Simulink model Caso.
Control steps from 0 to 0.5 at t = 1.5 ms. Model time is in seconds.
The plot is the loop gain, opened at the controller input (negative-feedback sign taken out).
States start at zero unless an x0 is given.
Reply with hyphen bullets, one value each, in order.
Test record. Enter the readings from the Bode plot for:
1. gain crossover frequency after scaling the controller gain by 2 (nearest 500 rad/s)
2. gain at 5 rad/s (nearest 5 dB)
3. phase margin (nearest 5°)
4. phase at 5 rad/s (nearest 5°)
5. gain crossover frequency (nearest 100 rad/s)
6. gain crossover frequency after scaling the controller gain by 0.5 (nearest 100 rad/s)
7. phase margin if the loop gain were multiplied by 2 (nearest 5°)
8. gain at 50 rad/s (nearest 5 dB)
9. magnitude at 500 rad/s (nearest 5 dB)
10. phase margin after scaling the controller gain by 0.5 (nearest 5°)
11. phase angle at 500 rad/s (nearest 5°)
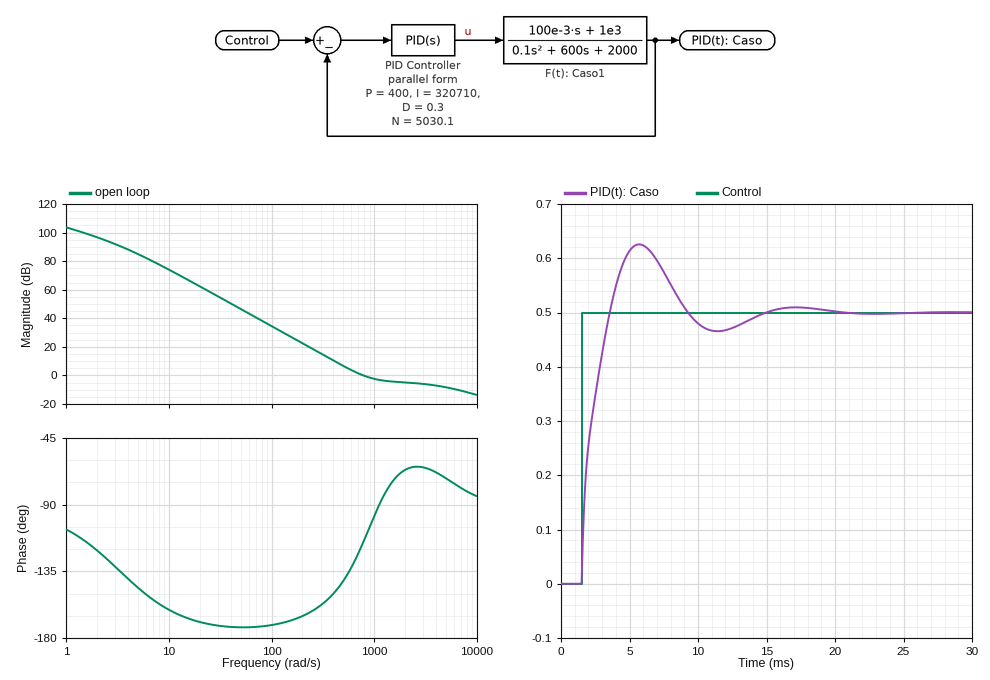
- 3000 rad/s
- 85 dB
- 65°
- -145°
- 800 rad/s
- 500 rad/s
- 115°
- 45 dB
- 5 dB
- 40°
- -140°
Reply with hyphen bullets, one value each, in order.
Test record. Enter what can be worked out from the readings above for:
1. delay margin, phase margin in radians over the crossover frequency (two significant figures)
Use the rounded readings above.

- 0.0014 s
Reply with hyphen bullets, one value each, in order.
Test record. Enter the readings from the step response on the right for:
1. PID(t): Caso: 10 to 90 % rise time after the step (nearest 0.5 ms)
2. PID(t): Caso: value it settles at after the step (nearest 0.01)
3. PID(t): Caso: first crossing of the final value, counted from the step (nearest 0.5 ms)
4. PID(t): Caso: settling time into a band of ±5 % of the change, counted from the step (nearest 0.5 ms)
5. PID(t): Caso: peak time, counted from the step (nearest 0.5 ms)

- 1.5 ms
- 0.50
- 2.0 ms
- 11.5 ms
- 4.0 ms
